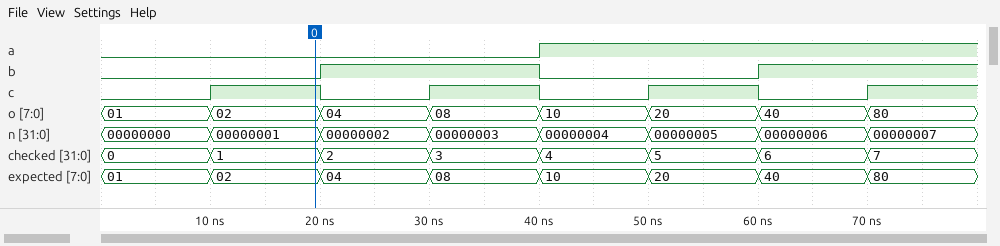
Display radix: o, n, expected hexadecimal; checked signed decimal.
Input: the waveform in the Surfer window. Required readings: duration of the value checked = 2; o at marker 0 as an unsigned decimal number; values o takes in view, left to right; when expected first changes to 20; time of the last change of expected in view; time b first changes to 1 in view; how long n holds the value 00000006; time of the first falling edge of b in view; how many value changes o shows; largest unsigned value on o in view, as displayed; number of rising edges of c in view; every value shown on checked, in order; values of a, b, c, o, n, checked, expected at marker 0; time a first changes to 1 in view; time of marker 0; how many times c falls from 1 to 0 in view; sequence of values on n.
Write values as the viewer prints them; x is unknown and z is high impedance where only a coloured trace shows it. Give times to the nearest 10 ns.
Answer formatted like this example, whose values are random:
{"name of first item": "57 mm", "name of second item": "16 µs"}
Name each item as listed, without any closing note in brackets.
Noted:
{"duration of the value checked = 2": "10 ns", "o at marker 0 as an unsigned decimal number": "2", "values o takes in view, left to right": "01, 02, 04, 08, 10, 20, 40, 80", "when expected first changes to 20": "50 ns", "time of the last change of expected in view": "70 ns", "time b first changes to 1 in view": "20 ns", "how long n holds the value 00000006": "10 ns", "time of the first falling edge of b in view": "40 ns", "how many value changes o shows": "7", "largest unsigned value on o in view, as displayed": "80", "number of rising edges of c in view": "4", "every value shown on checked, in order": "0, 1, 2, 3, 4, 5, 6, 7", "values of a, b, c, o, n, checked, expected at marker 0": "a=0, b=0, c=1, o=02, n=00000001, checked=1, expected=02", "time a first changes to 1 in view": "40 ns", "time of marker 0": "20 ns", "how many times c falls from 1 to 0 in view": "3", "sequence of values on n": "00000000, 00000001, 00000002, 00000003, 00000004, 00000005, 00000006, 00000007"}
